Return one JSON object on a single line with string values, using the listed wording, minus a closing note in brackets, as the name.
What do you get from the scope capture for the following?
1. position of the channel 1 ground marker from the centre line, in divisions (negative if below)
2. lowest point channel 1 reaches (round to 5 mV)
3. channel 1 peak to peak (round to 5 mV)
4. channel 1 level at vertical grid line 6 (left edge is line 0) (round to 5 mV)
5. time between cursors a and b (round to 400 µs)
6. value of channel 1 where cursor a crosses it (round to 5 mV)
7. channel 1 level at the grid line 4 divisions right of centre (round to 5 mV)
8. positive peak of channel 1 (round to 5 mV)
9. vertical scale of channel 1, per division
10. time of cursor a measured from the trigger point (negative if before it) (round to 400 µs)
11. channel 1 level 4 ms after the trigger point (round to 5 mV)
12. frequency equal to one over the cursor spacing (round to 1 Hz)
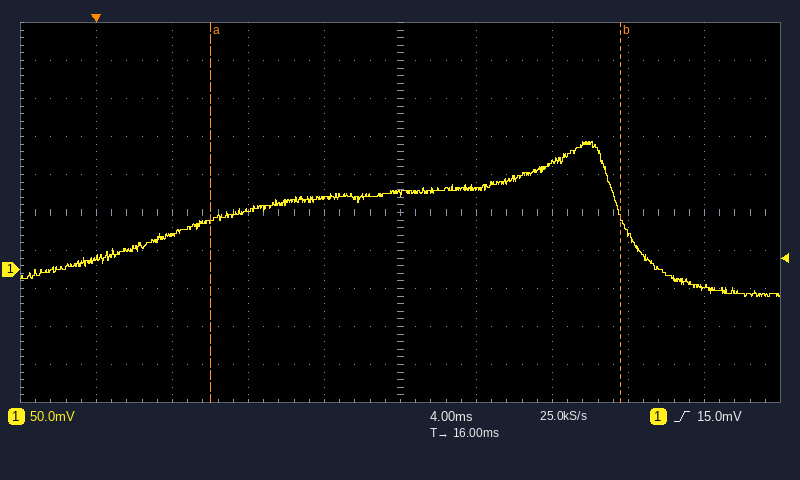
{"position of the channel 1 ground marker from the centre line, in divisions": "-1.5 div", "lowest point channel 1 reaches": "-35 mV", "channel 1 peak to peak": "205 mV", "channel 1 level at vertical grid line 6 (left edge is line 0)": "105 mV", "time between cursors a and b": "21.6 ms", "value of channel 1 where cursor a crosses it": "65 mV", "channel 1 level at the grid line 4 divisions right of centre": "-25 mV", "positive peak of channel 1": "170 mV", "vertical scale of channel 1, per division": "50 mV", "time of cursor a measured from the trigger point (negative if before it)": "+6.0 ms", "channel 1 level 4 ms after the trigger point": "45 mV", "frequency equal to one over the cursor spacing": "46 Hz"}
